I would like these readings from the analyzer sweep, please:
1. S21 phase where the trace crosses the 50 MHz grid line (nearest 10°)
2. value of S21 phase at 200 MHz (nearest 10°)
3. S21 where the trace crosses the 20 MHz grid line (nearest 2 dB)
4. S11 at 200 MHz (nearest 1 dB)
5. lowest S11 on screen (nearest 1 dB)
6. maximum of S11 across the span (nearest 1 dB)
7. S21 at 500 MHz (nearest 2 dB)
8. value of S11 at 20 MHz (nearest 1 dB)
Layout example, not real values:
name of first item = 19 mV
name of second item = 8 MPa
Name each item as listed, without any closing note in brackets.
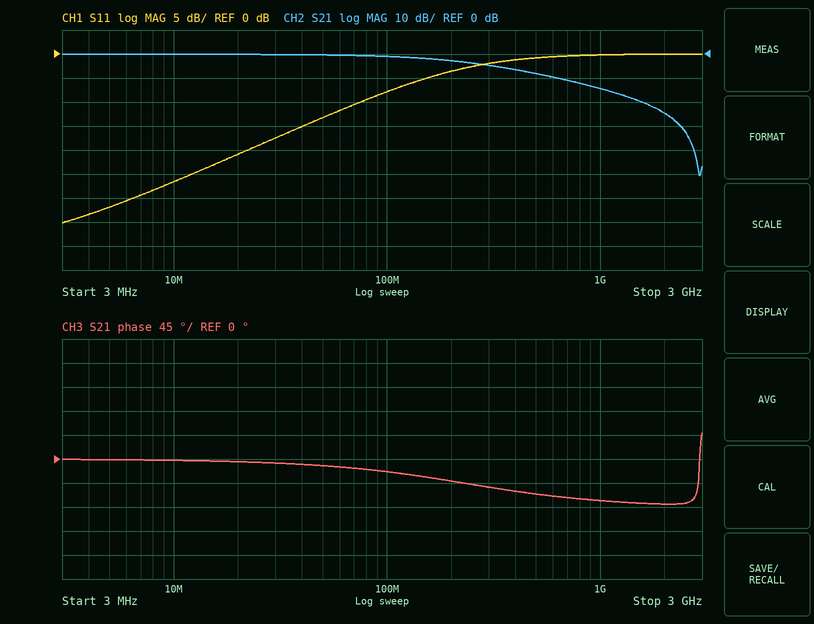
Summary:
S21 phase where the trace crosses the 50 MHz grid line = -10°
value of S21 phase at 200 MHz = -40°
S21 where the trace crosses the 20 MHz grid line = 0 dB
S11 at 200 MHz = -4 dB
lowest S11 on screen = -35 dB
maximum of S11 across the span = 0 dB
S21 at 500 MHz = -8 dB
value of S11 at 20 MHz = -21 dB
